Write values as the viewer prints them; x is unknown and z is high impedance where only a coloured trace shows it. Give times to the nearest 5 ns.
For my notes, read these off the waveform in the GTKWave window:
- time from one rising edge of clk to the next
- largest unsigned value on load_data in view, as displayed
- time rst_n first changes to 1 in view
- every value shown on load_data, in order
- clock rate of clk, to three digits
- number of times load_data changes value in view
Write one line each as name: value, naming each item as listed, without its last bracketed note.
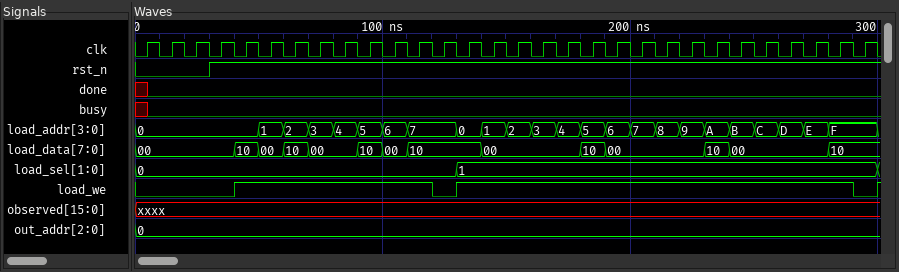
time from one rising edge of clk to the next: 10 ns
largest unsigned value on load_data in view, as displayed: 10
time rst_n first changes to 1 in view: 30 ns
every value shown on load_data, in order: 00, 10, 00, 10, 00, 10, 00, 10, 00, 10, 00, 10, 00, 10
clock rate of clk, to three digits: 100 MHz
number of times load_data changes value in view: 13
